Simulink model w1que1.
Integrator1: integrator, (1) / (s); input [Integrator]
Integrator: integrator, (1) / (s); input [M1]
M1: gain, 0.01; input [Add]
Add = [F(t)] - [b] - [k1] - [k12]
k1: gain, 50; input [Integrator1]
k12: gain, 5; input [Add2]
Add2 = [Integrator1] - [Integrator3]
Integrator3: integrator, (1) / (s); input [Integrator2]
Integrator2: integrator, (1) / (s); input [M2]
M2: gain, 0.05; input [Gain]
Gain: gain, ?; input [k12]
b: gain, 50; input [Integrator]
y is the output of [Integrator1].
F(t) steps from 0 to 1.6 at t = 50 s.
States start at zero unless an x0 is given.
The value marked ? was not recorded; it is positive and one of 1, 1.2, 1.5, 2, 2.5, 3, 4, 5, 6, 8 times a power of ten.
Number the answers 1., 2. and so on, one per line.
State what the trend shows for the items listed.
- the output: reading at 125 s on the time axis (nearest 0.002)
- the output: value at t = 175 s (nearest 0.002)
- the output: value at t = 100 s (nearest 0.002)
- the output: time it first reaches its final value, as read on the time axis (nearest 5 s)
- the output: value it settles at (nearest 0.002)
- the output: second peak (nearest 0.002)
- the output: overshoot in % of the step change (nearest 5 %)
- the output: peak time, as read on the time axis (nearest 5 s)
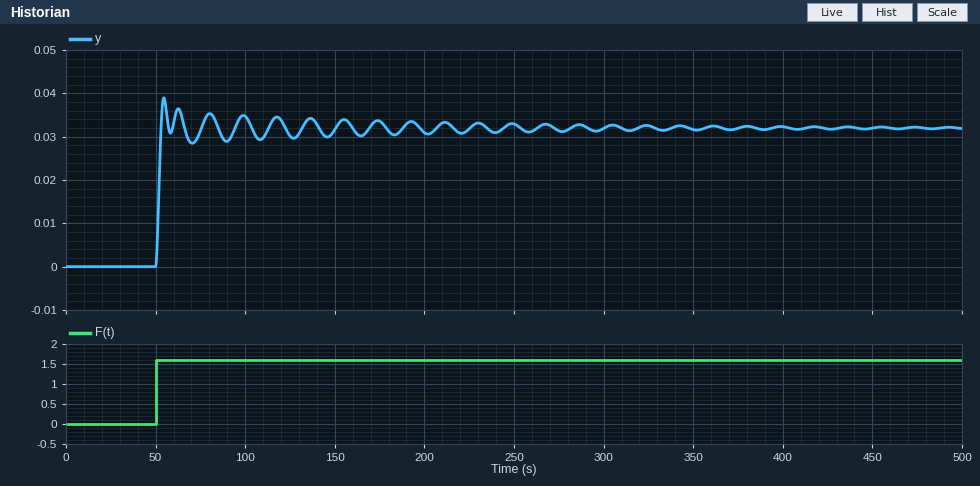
1. 0.030
2. 0.034
3. 0.034
4. 55 s
5. 0.032
6. 0.036
7. 20 %
8. 55 s
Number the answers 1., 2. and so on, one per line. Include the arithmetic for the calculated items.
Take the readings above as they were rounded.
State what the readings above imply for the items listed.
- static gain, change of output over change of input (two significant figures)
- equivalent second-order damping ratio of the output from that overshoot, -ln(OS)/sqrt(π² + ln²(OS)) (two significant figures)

1. (0.032 - 0) / (1.6 - 0) = 0.020
2. ln(0.2) = -1.609; 1.609 / sqrt(9.870 + 2.590) = 0.46
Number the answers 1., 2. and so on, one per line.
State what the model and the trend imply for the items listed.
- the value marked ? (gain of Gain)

1. 0.5
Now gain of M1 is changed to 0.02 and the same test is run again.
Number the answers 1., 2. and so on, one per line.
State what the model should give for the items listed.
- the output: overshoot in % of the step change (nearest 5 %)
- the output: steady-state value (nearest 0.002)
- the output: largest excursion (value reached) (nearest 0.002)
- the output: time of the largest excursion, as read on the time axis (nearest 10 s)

1. 10 %
2. 0.032
3. 0.036
4. 60 s
